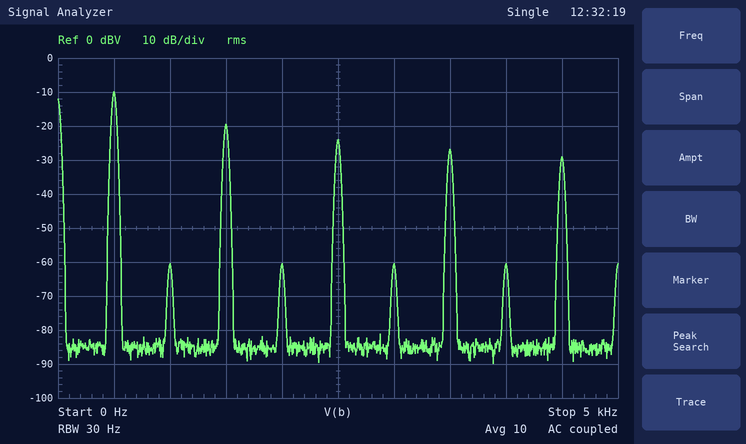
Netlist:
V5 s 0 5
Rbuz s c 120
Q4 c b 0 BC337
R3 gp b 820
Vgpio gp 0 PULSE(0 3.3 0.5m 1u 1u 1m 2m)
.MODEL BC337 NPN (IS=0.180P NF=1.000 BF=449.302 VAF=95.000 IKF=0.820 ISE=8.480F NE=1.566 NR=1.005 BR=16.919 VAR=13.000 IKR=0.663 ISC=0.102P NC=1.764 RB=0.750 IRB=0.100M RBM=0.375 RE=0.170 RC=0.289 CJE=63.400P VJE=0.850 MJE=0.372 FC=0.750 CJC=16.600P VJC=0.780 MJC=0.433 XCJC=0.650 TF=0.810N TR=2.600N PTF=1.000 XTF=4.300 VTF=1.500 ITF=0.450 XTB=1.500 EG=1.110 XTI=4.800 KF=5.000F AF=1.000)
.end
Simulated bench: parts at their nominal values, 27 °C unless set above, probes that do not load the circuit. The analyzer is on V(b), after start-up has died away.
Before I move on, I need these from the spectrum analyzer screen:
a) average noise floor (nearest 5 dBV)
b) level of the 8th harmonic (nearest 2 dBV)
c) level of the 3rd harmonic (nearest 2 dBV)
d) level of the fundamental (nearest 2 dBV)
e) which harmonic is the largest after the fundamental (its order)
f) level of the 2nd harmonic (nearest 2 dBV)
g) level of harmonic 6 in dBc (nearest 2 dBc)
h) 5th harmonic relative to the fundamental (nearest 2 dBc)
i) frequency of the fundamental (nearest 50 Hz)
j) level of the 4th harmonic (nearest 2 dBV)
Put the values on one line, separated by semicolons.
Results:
-85 dBV; -60 dBV; -20 dBV; -10 dBV; 3; -60 dBV; -50 dBc; -14 dBc; 500 Hz; -60 dBV
